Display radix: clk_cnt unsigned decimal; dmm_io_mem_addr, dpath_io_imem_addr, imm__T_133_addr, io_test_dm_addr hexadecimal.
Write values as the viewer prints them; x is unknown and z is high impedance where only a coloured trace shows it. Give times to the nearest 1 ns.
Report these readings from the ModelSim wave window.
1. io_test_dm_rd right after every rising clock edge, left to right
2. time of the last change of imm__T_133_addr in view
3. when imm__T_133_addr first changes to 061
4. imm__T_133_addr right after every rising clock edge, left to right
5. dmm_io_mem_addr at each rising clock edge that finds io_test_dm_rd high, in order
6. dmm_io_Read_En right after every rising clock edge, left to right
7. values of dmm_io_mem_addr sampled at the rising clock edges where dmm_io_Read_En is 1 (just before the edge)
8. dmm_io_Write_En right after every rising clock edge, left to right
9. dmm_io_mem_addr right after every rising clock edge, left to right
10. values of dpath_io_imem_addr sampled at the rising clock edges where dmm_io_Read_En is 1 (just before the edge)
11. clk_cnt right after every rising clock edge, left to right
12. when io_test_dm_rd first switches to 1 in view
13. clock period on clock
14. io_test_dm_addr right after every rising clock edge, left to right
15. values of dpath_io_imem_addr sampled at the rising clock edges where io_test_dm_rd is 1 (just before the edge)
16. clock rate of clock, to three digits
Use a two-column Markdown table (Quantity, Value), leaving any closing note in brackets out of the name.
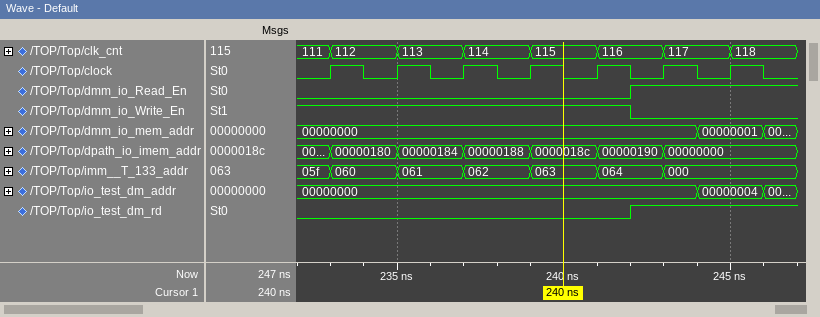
| Quantity | Value |
|---|---|
| io_test_dm_rd right after every rising clock edge, left to right | 0 0 0 0 0 1 1 |
| time of the last change of imm__T_133_addr in view | 243 ns |
| when imm__T_133_addr first changes to 061 | 235 ns |
| imm__T_133_addr right after every rising clock edge, left to right | 060, 061, 062, 063, 064, 000, 000 |
| dmm_io_mem_addr at each rising clock edge that finds io_test_dm_rd high, in order | 00000000, 00000001 |
| dmm_io_Read_En right after every rising clock edge, left to right | 0 0 0 0 0 1 1 |
| values of dmm_io_mem_addr sampled at the rising clock edges where dmm_io_Read_En is 1 | 00000000, 00000001 |
| dmm_io_Write_En right after every rising clock edge, left to right | 1 1 1 1 1 0 0 |
| dmm_io_mem_addr right after every rising clock edge, left to right | 00000000, 00000000, 00000000, 00000000, 00000000, 00000000, 00000001 |
| values of dpath_io_imem_addr sampled at the rising clock edges where dmm_io_Read_En is 1 | 00000190, 00000000 |
| clk_cnt right after every rising clock edge, left to right | 112, 113, 114, 115, 116, 117, 118 |
| when io_test_dm_rd first switches to 1 in view | 242 ns |
| clock period on clock | 2 ns |
| io_test_dm_addr right after every rising clock edge, left to right | 00000000, 00000000, 00000000, 00000000, 00000000, 00000000, 00000004 |
| values of dpath_io_imem_addr sampled at the rising clock edges where io_test_dm_rd is 1 | 00000190, 00000000 |
| clock rate of clock, to three digits | 500 MHz |
